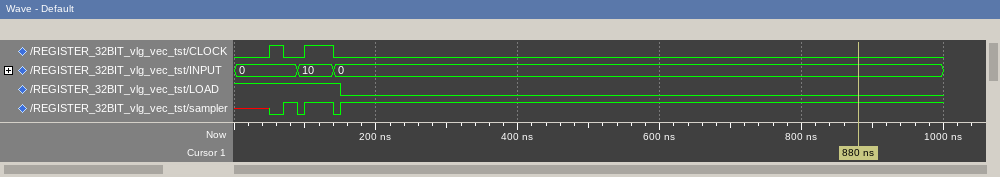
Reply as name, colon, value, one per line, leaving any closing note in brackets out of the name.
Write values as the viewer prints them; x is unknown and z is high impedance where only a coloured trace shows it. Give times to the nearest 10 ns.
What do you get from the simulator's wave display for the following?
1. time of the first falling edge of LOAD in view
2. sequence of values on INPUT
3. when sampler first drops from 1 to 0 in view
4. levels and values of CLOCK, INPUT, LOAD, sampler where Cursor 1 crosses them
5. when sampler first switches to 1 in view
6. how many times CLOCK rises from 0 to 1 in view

time of the first falling edge of LOAD in view: 150 ns
sequence of values on INPUT: 0, 10, 0
when sampler first drops from 1 to 0 in view: 90 ns
levels and values of CLOCK, INPUT, LOAD, sampler where Cursor 1 crosses them: CLOCK=0, INPUT=0, LOAD=0, sampler=1
when sampler first switches to 1 in view: 70 ns
how many times CLOCK rises from 0 to 1 in view: 2
